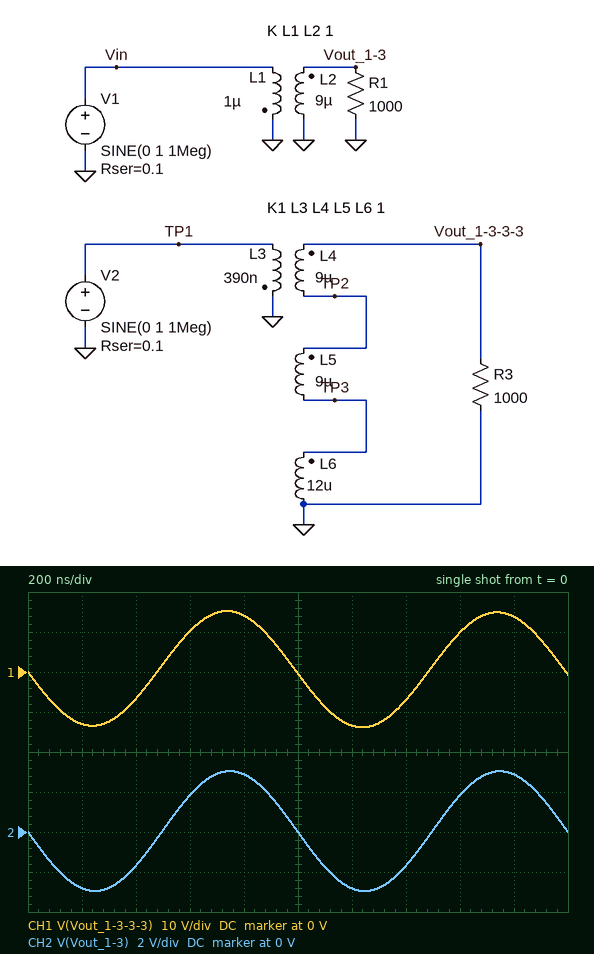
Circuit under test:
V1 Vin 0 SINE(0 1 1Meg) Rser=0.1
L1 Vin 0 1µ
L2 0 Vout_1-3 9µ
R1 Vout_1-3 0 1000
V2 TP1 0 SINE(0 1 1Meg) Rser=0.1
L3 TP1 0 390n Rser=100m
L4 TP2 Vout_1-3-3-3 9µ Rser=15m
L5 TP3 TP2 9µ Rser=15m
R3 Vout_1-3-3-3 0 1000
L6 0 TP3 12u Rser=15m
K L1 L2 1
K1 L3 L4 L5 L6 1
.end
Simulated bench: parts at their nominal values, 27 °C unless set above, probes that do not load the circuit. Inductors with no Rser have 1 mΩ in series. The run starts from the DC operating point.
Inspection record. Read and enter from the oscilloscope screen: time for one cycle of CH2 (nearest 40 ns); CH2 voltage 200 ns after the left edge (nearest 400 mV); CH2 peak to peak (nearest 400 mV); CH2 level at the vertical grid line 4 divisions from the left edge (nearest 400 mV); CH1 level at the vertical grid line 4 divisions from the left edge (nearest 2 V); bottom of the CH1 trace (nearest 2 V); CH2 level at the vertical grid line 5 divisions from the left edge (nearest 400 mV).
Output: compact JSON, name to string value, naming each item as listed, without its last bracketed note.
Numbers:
{"time for one cycle of CH2": "1.00 µs", "CH2 voltage 200 ns after the left edge": "-2.8 V", "CH2 peak to peak": "6.0 V", "CH2 level at the vertical grid line 4 divisions from the left edge": "2.8 V", "CH1 level at the vertical grid line 4 divisions from the left edge": "14 V", "bottom of the CH1 trace": "-14 V", "CH2 level at the vertical grid line 5 divisions from the left edge": "0 V"}
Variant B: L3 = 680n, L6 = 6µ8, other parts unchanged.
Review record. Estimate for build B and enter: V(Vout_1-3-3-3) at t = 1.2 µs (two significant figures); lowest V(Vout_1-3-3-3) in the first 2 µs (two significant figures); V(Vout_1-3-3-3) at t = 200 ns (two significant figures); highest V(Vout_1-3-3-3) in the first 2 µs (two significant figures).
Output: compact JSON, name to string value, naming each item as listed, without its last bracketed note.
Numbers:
{"V(Vout_1-3-3-3) at t = 1.2 µs": "-9.5 V", "lowest V(Vout_1-3-3-3) in the first 2 µs": "-9.9 V", "V(Vout_1-3-3-3) at t = 200 ns": "-9.4 V", "highest V(Vout_1-3-3-3) in the first 2 µs": "11 V"}
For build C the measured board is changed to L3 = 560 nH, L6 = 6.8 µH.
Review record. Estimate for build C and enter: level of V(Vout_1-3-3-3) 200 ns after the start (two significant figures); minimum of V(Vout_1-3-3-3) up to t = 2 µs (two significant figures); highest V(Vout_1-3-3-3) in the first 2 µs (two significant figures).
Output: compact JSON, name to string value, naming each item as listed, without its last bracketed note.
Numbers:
{"level of V(Vout_1-3-3-3) 200 ns after the start": "-10 V", "minimum of V(Vout_1-3-3-3) up to t = 2 µs": "-11 V", "highest V(Vout_1-3-3-3) in the first 2 µs": "12 V"}
